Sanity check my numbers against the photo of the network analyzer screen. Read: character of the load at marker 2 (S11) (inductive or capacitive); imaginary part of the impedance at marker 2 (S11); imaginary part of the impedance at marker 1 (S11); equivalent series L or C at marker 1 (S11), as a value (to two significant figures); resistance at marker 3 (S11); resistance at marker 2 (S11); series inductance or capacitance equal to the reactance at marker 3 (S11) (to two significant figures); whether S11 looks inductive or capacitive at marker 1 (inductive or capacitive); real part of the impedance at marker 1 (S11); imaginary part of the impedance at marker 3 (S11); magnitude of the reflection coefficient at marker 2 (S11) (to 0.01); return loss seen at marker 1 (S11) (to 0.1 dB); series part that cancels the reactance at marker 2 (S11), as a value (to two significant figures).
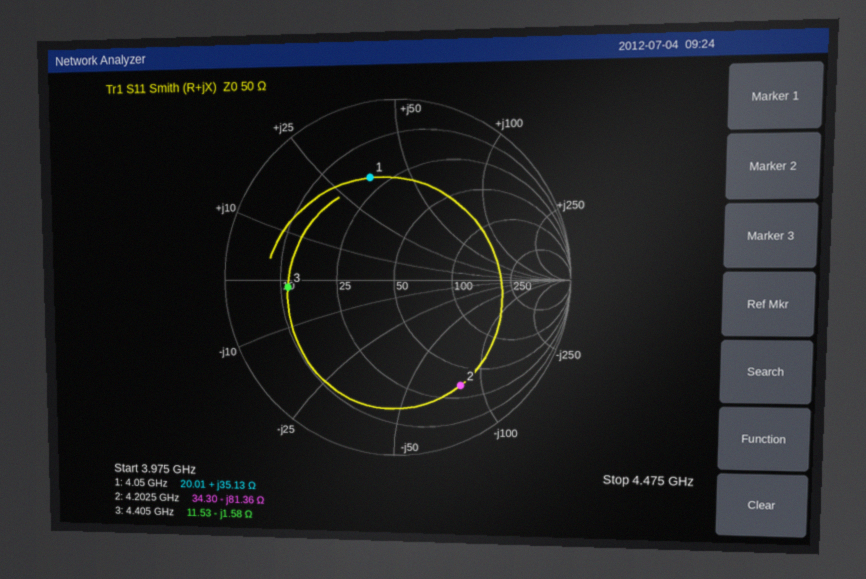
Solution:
capacitive
-81.36 Ω
+35.13 Ω
1.4 nH
11.53 Ω
34.30 Ω
23 pF
inductive
20.01 Ω
-1.58 Ω
0.71
4.6 dB
3.1 nH
